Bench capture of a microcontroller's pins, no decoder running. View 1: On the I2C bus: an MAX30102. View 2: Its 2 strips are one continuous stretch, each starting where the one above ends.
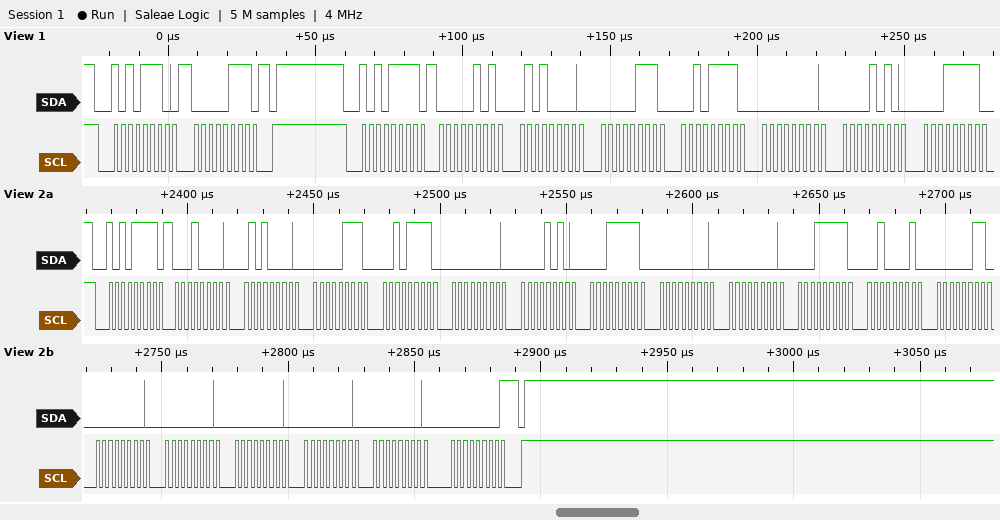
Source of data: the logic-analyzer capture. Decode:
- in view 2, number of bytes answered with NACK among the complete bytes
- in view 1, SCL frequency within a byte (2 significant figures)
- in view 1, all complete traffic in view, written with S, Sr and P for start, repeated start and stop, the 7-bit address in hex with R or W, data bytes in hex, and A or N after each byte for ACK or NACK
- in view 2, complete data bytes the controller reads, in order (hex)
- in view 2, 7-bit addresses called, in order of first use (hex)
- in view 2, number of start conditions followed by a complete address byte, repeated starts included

1
400 kHz
S 57W A 07 A P S 57R A 05 A 50 A 07 A 2F A 00 A 0A A 1F A
10 50 07 2F 00 0A 1F 00 00 1F 21 03 00 00 00 00 00 00
0x57
1
